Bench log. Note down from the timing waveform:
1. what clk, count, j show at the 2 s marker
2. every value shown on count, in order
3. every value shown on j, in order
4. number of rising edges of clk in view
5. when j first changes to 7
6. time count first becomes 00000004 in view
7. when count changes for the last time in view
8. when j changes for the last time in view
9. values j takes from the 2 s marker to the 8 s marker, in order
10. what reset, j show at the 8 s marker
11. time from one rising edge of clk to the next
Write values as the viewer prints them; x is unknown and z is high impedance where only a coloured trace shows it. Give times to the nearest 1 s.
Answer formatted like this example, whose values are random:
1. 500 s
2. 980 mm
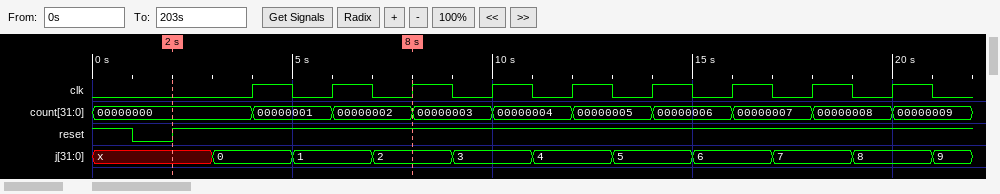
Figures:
1. clk=0, count=00000000, j=x
2. 00000000, 00000001, 00000002, 00000003, 00000004, 00000005, 00000006, 00000007, 00000008, 00000009
3. x, 0, 1, 2, 3, 4, 5, 6, 7, 8, 9
4. 9
5. 17 s
6. 10 s
7. 20 s
8. 21 s
9. x, 0, 1, 2
10. reset=1, j=2
11. 2 s
